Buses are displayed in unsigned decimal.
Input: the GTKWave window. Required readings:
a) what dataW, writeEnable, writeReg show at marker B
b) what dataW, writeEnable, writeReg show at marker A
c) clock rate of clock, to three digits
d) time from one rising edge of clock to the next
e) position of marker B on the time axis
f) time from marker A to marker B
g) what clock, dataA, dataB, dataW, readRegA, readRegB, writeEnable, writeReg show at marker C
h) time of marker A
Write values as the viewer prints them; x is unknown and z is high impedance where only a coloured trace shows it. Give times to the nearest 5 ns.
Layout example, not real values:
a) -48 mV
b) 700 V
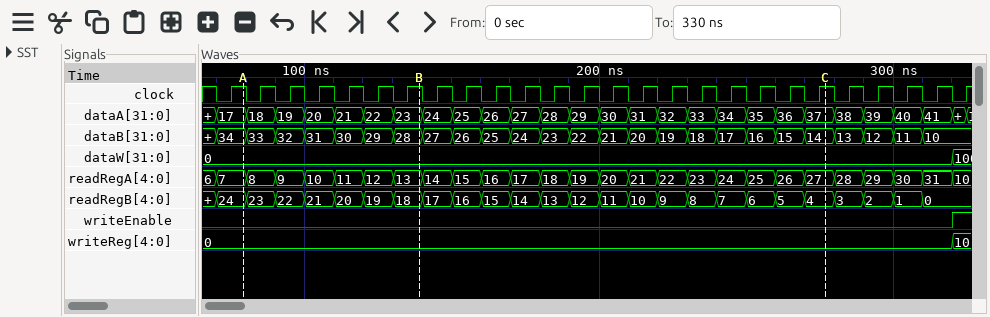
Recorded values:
a) dataW=0, writeEnable=0, writeReg=0
b) dataW=0, writeEnable=0, writeReg=0
c) 100 MHz
d) 10 ns
e) 140 ns
f) 60 ns
g) clock=1, dataA=37, dataB=14, dataW=0, readRegA=27, readRegB=4, writeEnable=0, writeReg=0
h) 80 ns
